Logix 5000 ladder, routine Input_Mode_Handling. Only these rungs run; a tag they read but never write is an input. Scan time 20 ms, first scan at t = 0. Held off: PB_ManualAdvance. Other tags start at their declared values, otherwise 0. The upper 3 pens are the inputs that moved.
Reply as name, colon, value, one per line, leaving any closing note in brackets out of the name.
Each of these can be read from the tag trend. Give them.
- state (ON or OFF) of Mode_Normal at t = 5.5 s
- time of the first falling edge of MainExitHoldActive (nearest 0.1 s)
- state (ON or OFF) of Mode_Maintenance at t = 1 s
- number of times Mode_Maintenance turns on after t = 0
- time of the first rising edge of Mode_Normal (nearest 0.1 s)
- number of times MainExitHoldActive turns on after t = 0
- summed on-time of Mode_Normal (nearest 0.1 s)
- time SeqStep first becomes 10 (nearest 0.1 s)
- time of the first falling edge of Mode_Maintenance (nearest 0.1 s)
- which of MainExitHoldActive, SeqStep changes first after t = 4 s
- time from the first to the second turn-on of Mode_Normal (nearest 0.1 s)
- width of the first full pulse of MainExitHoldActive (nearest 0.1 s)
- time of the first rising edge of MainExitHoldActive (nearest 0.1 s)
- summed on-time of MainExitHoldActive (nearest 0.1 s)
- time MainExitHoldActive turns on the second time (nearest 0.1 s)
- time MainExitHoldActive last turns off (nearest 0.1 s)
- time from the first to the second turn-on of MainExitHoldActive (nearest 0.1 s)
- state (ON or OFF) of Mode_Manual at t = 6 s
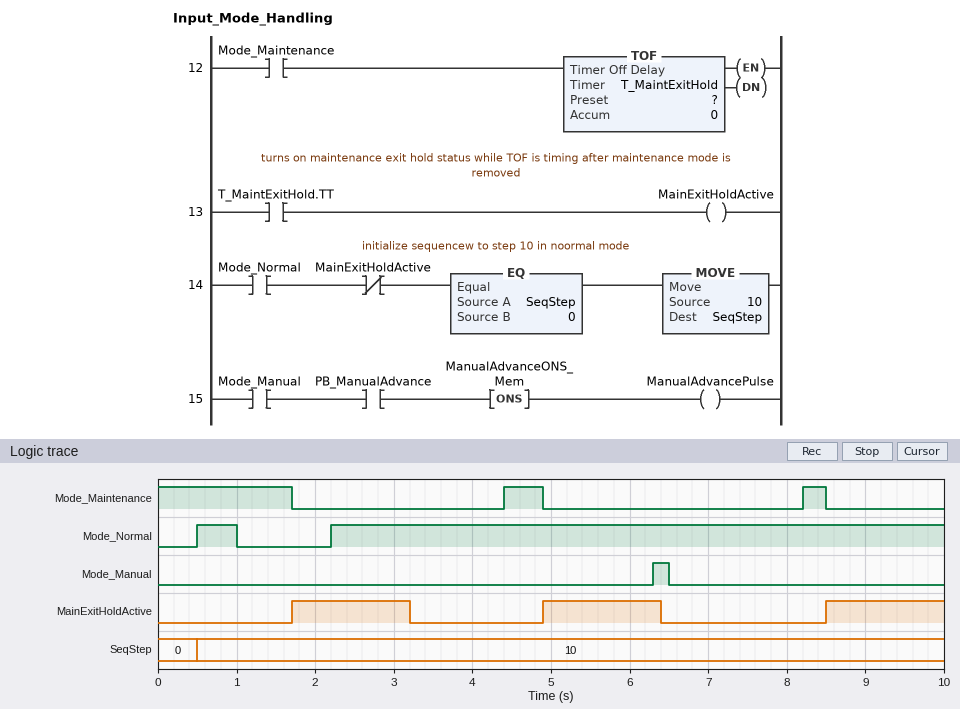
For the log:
state (ON or OFF) of Mode_Normal at t = 5.5 s: ON
time of the first falling edge of MainExitHoldActive: 3.2 s
state (ON or OFF) of Mode_Maintenance at t = 1 s: ON
number of times Mode_Maintenance turns on after t = 0: 2
time of the first rising edge of Mode_Normal: 0.5 s
number of times MainExitHoldActive turns on after t = 0: 3
summed on-time of Mode_Normal: 8.3 s
time SeqStep first becomes 10: 0.5 s
time of the first falling edge of Mode_Maintenance: 1.7 s
which of MainExitHoldActive, SeqStep changes first after t = 4 s: MainExitHoldActive
time from the first to the second turn-on of Mode_Normal: 1.7 s
width of the first full pulse of MainExitHoldActive: 1.5 s
time of the first rising edge of MainExitHoldActive: 1.7 s
summed on-time of MainExitHoldActive: 4.5 s
time MainExitHoldActive turns on the second time: 4.9 s
time MainExitHoldActive last turns off: 6.4 s
time from the first to the second turn-on of MainExitHoldActive: 3.2 s
state (ON or OFF) of Mode_Manual at t = 6 s: OFF
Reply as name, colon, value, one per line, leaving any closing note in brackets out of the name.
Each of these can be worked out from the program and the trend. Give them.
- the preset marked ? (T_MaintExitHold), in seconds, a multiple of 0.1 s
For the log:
the preset marked ? (T_MaintExitHold), in seconds, a multiple of 0.1 s: 1.5 s
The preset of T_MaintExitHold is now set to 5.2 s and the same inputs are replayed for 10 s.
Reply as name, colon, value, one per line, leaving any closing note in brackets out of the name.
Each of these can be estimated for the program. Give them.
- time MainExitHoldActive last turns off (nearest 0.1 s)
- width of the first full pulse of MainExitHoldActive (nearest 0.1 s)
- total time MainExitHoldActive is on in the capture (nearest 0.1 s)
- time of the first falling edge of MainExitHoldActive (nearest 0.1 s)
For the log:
time MainExitHoldActive last turns off: 8.2 s
width of the first full pulse of MainExitHoldActive: 2.7 s
total time MainExitHoldActive is on in the capture: 7.5 s
time of the first falling edge of MainExitHoldActive: 4.4 s
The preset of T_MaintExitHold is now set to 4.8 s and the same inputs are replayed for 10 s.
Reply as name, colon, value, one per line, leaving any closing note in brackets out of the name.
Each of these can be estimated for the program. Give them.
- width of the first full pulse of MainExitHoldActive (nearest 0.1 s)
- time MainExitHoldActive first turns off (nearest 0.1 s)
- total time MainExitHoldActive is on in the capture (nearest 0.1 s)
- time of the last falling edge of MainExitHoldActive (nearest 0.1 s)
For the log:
width of the first full pulse of MainExitHoldActive: 2.7 s
time MainExitHoldActive first turns off: 4.4 s
total time MainExitHoldActive is on in the capture: 7.5 s
time of the last falling edge of MainExitHoldActive: 8.2 s
